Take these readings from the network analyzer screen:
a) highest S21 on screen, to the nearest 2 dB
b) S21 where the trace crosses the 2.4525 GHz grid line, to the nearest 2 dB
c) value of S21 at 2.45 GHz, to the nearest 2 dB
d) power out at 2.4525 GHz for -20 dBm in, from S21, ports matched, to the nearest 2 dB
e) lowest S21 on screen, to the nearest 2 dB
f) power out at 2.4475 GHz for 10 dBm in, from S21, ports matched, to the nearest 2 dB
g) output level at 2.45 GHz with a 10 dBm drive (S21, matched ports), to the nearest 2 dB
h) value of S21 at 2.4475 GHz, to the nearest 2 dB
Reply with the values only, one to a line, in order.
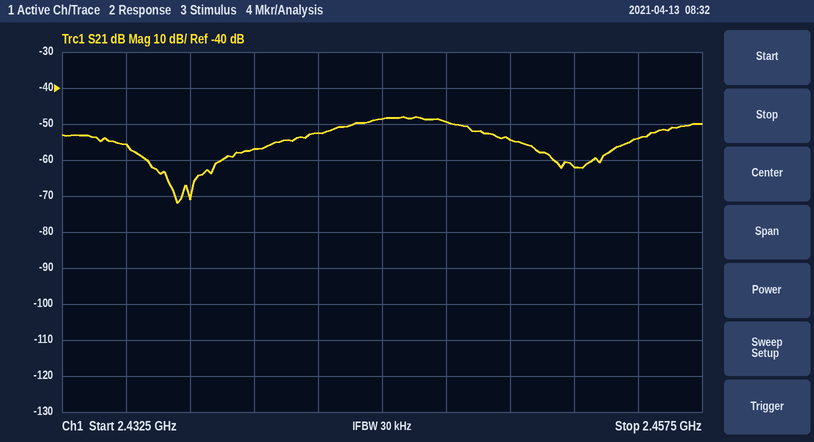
-48 dB
-62 dB
-54 dB
-82 dBm
-72 dB
-40 dBm
-44 dBm
-50 dB
